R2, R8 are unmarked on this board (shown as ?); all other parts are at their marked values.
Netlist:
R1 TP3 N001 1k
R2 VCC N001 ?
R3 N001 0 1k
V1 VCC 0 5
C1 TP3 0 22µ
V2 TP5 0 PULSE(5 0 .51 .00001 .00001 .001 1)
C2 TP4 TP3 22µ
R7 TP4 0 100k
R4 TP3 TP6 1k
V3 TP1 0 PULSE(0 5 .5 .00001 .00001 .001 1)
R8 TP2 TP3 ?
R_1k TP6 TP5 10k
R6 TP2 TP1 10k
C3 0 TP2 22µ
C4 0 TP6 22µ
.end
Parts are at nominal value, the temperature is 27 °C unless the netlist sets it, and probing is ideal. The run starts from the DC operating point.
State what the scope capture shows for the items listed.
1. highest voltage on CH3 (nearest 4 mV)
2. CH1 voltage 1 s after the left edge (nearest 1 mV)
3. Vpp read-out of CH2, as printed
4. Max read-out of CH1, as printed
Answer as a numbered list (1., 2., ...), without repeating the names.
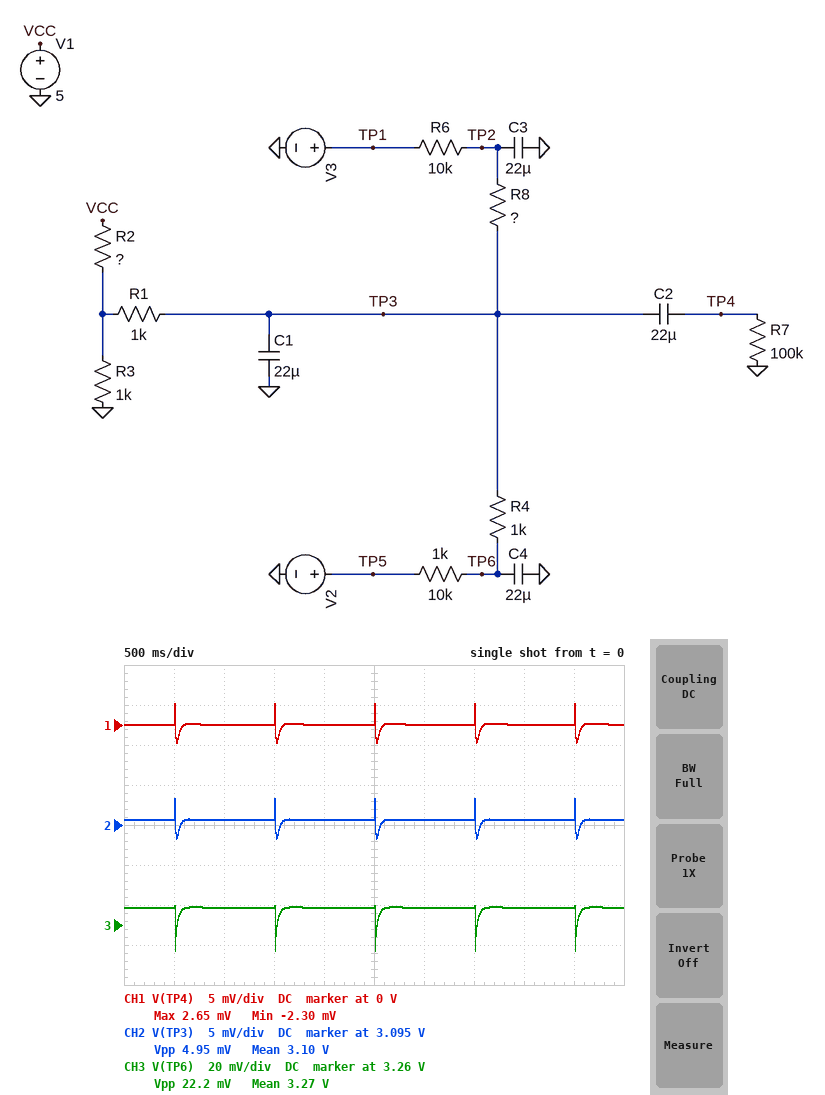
1. 3.268 V
2. 0 V
3. 4.95 mV
4. 2.65 mV
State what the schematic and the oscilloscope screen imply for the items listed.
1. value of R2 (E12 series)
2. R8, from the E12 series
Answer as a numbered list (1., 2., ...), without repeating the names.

1. 560 Ω
2. 2.2 kΩ
